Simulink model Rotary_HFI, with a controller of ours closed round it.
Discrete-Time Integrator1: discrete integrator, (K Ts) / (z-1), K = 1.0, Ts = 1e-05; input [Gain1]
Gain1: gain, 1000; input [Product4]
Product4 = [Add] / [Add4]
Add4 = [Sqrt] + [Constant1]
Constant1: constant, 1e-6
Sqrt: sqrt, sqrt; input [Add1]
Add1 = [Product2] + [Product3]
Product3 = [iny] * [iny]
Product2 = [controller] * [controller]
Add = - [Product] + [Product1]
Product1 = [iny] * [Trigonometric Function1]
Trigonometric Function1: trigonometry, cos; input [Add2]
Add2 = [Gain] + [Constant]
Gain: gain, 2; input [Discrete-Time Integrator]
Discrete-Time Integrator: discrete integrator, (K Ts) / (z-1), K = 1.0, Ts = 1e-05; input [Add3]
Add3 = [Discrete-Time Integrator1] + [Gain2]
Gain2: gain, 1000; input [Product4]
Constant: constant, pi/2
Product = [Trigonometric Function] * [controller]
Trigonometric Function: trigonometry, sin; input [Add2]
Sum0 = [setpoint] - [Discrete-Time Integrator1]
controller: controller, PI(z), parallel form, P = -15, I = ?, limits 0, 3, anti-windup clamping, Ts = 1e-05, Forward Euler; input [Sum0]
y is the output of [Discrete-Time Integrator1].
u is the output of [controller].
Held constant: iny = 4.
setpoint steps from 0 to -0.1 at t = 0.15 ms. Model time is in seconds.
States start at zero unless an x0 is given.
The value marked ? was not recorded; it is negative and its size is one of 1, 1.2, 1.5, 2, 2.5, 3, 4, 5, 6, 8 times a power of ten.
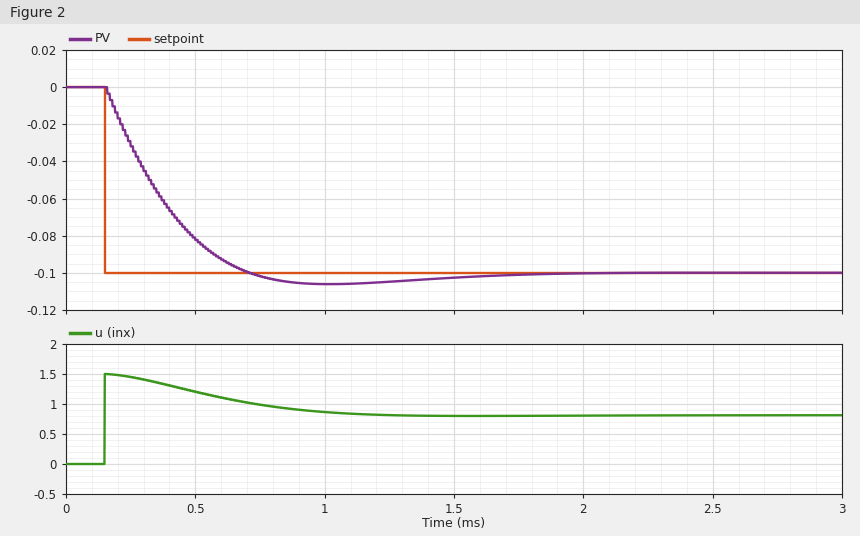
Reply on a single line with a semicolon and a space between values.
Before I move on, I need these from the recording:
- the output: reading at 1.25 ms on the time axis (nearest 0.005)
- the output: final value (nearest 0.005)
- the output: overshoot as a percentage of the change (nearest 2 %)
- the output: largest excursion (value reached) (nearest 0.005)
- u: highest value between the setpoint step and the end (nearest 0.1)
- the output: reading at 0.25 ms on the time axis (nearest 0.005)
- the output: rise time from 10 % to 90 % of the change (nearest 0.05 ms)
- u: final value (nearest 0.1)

-0.105; -0.100; 6 %; -0.105; 1.5; -0.030; 0.40 ms; 0.8
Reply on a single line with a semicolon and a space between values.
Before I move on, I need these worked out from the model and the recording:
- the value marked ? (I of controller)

-50000
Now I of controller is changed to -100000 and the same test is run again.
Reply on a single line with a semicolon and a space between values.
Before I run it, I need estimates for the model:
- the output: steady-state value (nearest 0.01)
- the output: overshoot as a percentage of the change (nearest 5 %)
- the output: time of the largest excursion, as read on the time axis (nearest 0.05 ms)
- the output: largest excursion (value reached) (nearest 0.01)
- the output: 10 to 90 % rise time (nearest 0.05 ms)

-0.10; 20 %; 0.75 ms; -0.12; 0.25 ms
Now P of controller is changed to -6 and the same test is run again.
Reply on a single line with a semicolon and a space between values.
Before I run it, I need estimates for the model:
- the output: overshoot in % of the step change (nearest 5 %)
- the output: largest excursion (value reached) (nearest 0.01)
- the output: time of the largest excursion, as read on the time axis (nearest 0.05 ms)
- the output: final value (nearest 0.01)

20 %; -0.12; 1.05 ms; -0.10
